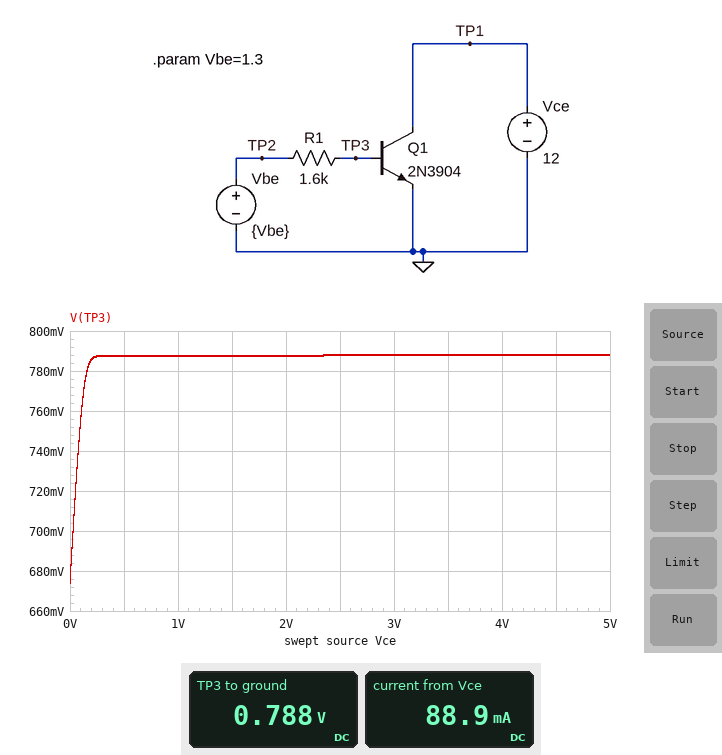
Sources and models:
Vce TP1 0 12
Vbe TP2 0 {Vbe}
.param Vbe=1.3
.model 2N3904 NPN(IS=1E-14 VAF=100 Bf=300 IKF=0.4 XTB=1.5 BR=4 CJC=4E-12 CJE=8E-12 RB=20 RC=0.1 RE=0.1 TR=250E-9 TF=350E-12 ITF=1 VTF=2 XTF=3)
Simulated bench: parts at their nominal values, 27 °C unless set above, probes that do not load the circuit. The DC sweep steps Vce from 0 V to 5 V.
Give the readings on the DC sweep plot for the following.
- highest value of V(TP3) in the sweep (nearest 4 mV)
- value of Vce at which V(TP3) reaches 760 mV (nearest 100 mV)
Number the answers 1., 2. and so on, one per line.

1. 788 mV
2. 100 mV
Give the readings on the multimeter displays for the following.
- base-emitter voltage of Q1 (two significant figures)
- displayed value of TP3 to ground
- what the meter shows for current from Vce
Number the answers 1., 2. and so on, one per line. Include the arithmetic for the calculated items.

1. 788 mV = 790 mV
2. 0.788 V
3. 88.9 mA
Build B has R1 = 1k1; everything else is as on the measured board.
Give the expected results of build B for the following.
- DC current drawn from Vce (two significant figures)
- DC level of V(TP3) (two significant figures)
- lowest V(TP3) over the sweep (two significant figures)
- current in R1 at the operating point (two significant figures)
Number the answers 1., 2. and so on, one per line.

1. 120 mA
2. 800 mV
3. 690 mV
4. 450 µA
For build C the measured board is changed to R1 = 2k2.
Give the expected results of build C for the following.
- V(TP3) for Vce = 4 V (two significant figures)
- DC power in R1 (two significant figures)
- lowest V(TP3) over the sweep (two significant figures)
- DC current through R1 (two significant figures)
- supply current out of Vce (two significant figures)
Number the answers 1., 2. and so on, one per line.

1. 780 mV
2. 120 µW
3. 660 mV
4. 240 µA
5. 69 mA
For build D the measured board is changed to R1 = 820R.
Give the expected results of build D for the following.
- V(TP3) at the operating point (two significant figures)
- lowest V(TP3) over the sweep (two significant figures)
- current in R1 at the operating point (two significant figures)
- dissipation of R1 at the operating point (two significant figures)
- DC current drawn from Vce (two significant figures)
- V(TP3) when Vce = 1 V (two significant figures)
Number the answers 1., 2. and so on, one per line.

1. 820 mV
2. 700 mV
3. 590 µA
4. 290 µW
5. 150 mA
6. 810 mV
